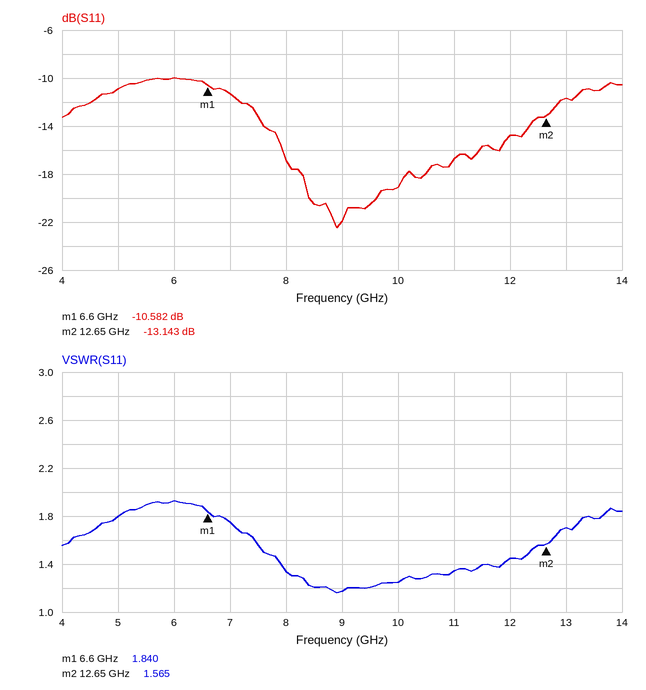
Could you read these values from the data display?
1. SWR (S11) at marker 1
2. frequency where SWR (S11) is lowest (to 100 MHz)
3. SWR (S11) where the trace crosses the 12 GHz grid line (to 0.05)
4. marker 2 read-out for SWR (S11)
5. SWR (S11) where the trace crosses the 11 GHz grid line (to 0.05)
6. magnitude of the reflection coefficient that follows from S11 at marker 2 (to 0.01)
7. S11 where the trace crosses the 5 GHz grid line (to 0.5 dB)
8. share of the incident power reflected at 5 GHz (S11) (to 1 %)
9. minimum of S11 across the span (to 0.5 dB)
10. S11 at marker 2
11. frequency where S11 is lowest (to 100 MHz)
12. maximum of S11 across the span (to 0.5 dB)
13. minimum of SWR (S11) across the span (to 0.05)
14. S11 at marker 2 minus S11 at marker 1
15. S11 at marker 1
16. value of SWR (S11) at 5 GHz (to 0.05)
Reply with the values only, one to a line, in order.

1.840
8.9 GHz
1.45
1.565
1.35
0.22
-11.0 dB
8 %
-22.5 dB
-13.143 dB
8.9 GHz
-10.0 dB
1.15
-2.561 dB
-10.582 dB
1.80
